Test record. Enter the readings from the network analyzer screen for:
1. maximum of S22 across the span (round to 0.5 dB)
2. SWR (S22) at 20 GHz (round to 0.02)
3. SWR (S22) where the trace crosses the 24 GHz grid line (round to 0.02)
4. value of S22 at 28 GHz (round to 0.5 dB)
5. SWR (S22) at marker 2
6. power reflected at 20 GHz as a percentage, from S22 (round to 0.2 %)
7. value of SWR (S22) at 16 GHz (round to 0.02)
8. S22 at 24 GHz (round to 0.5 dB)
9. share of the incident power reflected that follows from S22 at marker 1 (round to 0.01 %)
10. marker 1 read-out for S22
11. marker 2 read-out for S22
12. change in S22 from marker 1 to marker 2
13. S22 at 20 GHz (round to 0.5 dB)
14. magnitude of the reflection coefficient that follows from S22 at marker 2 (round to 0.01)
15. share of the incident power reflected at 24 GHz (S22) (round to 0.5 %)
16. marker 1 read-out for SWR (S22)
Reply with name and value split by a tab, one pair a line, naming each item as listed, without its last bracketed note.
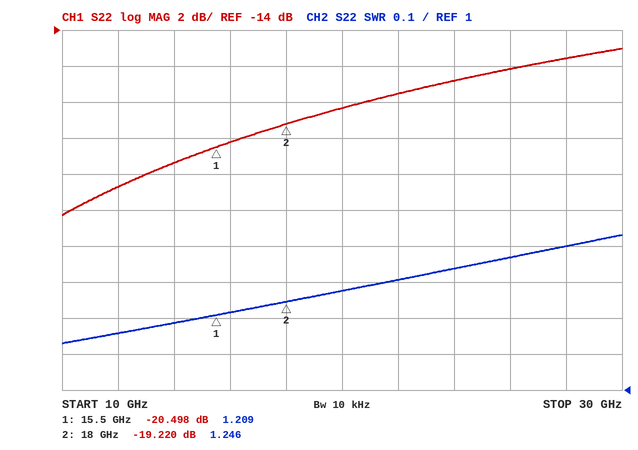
maximum of S22 across the span	-15.0 dB
SWR (S22) at 20 GHz	1.28
SWR (S22) where the trace crosses the 24 GHz grid line	1.34
value of S22 at 28 GHz	-15.5 dB
SWR (S22) at marker 2	1.246
power reflected at 20 GHz as a percentage, from S22	1.4 %
value of SWR (S22) at 16 GHz	1.22
S22 at 24 GHz	-17.0 dB
share of the incident power reflected that follows from S22 at marker 1	0.89 %
marker 1 read-out for S22	-20.498 dB
marker 2 read-out for S22	-19.220 dB
change in S22 from marker 1 to marker 2	1.278 dB
S22 at 20 GHz	-18.5 dB
magnitude of the reflection coefficient that follows from S22 at marker 2	0.11
share of the incident power reflected at 24 GHz (S22)	2.0 %
marker 1 read-out for SWR	1.209
